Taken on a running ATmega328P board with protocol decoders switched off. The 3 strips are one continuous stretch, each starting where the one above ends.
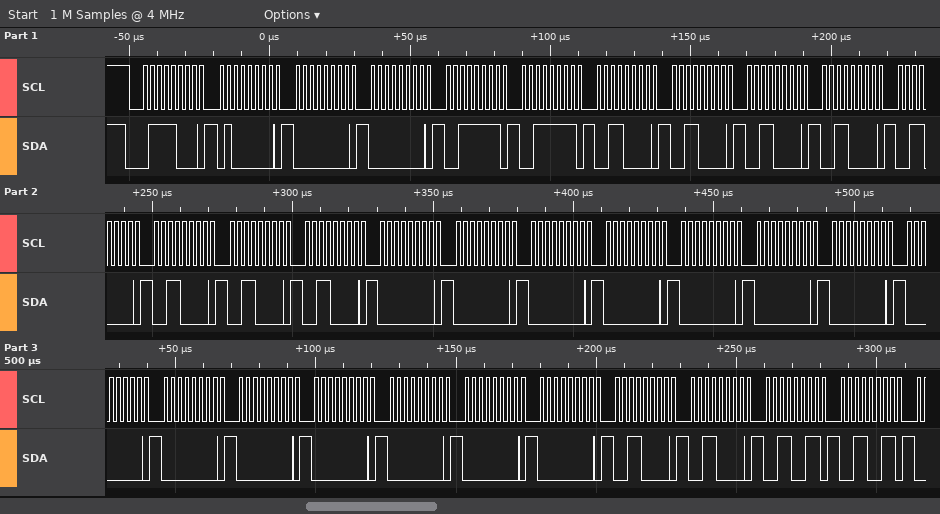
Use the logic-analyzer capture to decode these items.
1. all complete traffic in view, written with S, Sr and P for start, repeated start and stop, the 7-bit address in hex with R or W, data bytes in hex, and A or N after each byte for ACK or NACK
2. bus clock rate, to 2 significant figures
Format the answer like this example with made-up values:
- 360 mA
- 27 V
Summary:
- S 3CW A 40 A 00 A 00 A 3F A 3F A 30 A 30 A 30 A 30 A 30 A 30 A 30 A 30 A 00 A 00 A 00 A 00 A 00 A 00 A 00 A 00 A 00 A 00 A 00 A 00 A 00 A 00 A 30 A 30 A 33 A 33 A
- 400 kHz
